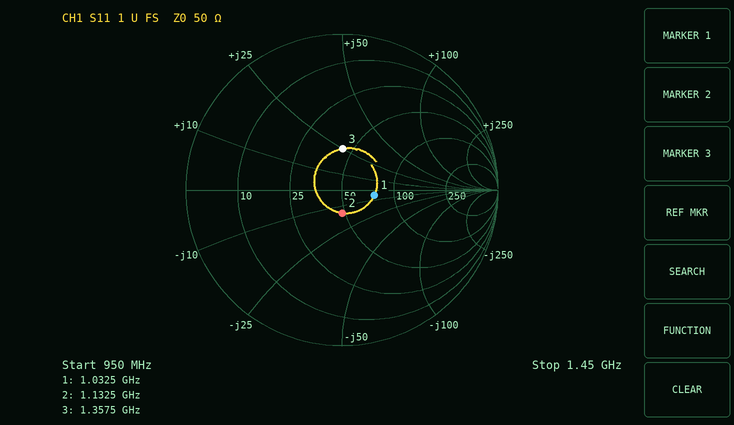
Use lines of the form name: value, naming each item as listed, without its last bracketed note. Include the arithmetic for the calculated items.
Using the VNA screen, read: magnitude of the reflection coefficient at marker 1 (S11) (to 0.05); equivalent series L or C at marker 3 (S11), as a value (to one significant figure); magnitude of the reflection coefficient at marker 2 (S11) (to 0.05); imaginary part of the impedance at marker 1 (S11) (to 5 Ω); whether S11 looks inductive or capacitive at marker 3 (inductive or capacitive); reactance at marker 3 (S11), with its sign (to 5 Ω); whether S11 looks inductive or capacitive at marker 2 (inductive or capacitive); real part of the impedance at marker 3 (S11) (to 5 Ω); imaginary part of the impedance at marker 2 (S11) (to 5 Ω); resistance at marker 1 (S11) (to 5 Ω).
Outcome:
magnitude of the reflection coefficient at marker 1 (S11): 0.20
equivalent series L or C at marker 3 (S11), as a value: L = 25 Ω/(2π × 1.3575 GHz) ≈ 3 nH
magnitude of the reflection coefficient at marker 2 (S11): 0.15
imaginary part of the impedance at marker 1 (S11): -5 Ω
whether S11 looks inductive or capacitive at marker 3: inductive
reactance at marker 3 (S11), with its sign: +25 Ω
whether S11 looks inductive or capacitive at marker 2: capacitive
real part of the impedance at marker 3 (S11): 45 Ω
imaginary part of the impedance at marker 2 (S11): -15 Ω
resistance at marker 1 (S11): 75 Ω
